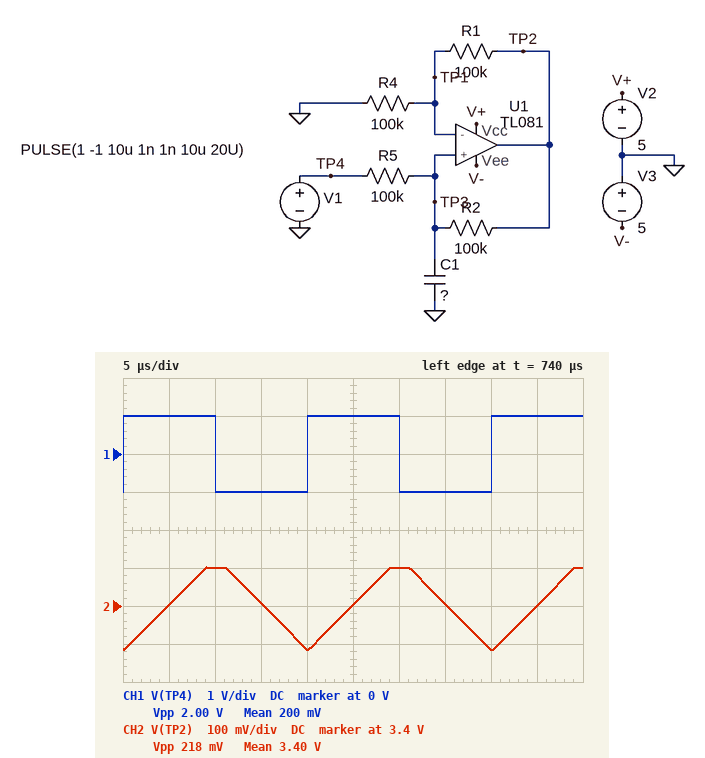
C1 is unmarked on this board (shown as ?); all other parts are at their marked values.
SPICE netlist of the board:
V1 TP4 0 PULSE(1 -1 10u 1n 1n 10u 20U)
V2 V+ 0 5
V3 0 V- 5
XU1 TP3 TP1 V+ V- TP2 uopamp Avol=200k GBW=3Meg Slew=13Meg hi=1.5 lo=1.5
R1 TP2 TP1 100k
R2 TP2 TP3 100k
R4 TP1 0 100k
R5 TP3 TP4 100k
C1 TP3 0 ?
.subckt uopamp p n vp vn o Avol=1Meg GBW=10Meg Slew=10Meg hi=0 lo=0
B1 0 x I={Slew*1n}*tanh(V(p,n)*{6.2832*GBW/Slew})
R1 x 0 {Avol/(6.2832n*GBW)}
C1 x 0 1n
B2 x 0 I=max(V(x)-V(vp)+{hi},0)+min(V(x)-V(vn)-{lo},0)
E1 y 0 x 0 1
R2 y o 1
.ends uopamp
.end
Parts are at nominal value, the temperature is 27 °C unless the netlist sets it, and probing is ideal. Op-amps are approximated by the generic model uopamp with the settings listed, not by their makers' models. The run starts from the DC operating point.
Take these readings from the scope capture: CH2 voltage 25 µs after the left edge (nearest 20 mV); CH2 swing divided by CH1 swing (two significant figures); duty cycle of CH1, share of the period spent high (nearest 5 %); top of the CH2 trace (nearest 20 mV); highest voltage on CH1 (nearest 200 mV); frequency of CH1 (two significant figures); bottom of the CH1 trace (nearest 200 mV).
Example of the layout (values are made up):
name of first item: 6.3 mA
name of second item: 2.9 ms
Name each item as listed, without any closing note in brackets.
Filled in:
CH2 voltage 25 µs after the left edge: 3.40 V
CH2 swing divided by CH1 swing: 0.11
duty cycle of CH1, share of the period spent high: 50 %
top of the CH2 trace: 3.50 V
highest voltage on CH1: 1.0 V
frequency of CH1: 50 kHz
bottom of the CH1 trace: -1.0 V
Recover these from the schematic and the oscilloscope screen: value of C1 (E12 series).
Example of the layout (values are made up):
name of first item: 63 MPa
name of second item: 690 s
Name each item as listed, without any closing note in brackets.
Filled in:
value of C1: 820 pF
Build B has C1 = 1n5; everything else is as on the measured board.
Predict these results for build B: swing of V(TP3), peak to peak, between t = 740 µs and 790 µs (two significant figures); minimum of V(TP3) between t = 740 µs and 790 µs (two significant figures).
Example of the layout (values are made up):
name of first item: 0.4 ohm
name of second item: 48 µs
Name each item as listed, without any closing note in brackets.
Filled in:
swing of V(TP3), peak to peak, between t = 740 µs and 790 µs: 67 mV
minimum of V(TP3) between t = 740 µs and 790 µs: 1.7 V
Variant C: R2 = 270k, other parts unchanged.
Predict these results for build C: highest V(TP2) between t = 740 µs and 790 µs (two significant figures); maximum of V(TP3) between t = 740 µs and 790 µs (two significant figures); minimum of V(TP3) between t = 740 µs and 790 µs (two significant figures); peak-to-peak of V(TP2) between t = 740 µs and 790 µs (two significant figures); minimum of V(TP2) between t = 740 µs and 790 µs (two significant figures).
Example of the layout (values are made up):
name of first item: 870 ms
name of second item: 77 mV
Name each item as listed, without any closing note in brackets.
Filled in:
highest V(TP2) between t = 740 µs and 790 µs: 130 mV
maximum of V(TP3) between t = 740 µs and 790 µs: 66 mV
minimum of V(TP3) between t = 740 µs and 790 µs: -57 mV
peak-to-peak of V(TP2) between t = 740 µs and 790 µs: 240 mV
minimum of V(TP2) between t = 740 µs and 790 µs: -110 mV
